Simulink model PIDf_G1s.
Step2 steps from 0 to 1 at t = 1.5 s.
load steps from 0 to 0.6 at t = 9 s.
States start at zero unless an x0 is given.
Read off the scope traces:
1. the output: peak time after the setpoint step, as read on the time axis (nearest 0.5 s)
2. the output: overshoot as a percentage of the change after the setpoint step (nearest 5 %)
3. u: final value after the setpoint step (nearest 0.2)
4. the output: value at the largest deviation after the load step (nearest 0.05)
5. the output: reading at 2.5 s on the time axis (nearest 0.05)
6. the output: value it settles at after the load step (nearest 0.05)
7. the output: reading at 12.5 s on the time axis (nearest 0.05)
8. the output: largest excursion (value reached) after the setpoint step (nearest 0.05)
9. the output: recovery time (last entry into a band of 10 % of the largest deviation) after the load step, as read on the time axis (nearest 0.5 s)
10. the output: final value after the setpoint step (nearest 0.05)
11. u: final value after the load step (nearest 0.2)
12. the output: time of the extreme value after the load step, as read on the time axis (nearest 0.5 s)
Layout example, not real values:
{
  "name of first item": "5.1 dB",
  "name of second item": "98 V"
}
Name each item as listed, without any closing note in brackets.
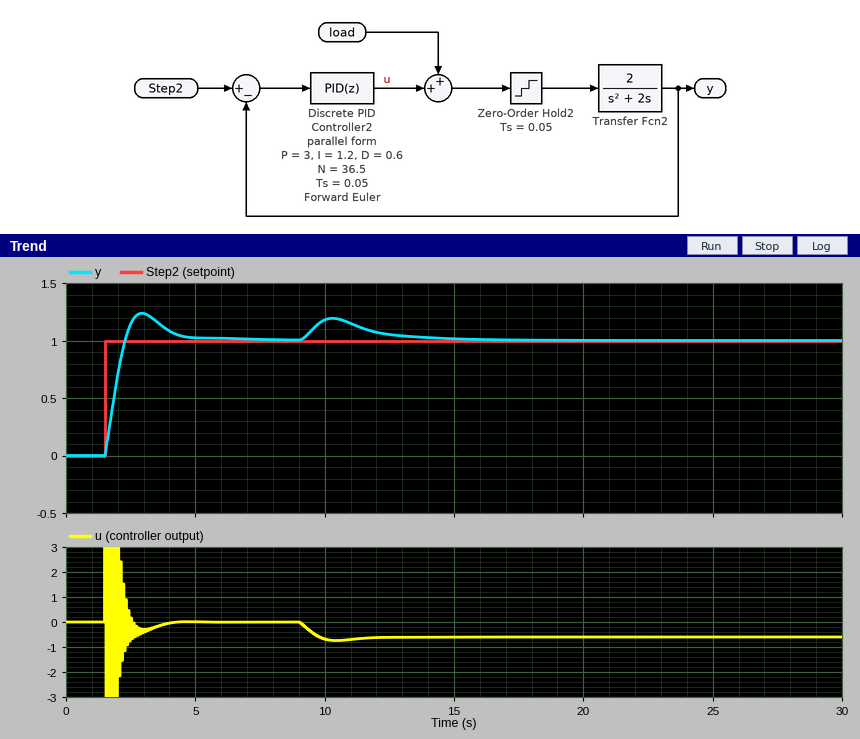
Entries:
{
  "the output: peak time after the setpoint step, as read on the time axis": "3.0 s",
  "the output: overshoot as a percentage of the change after the setpoint step": "25 %",
  "u: final value after the setpoint step": "0.0",
  "the output: value at the largest deviation after the load step": "1.20",
  "the output: reading at 2.5 s on the time axis": "1.15",
  "the output: value it settles at after the load step": "1.00",
  "the output: reading at 12.5 s on the time axis": "1.05",
  "the output: largest excursion (value reached) after the setpoint step": "1.25",
  "the output: recovery time (last entry into a band of 10 % of the largest deviation) after the load step, as read on the time axis": "14.5 s",
  "the output: final value after the setpoint step": "1.00",
  "u: final value after the load step": "-0.6",
  "the output: time of the extreme value after the load step, as read on the time axis": "10.5 s"
}
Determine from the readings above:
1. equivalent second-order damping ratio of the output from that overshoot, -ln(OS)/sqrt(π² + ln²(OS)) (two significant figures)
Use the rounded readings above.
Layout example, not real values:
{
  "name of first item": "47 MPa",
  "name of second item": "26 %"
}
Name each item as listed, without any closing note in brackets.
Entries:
{
  "equivalent second-order damping ratio of the output from that overshoot, -ln(OS)/sqrt(π² + ln²(OS))": "0.40"
}
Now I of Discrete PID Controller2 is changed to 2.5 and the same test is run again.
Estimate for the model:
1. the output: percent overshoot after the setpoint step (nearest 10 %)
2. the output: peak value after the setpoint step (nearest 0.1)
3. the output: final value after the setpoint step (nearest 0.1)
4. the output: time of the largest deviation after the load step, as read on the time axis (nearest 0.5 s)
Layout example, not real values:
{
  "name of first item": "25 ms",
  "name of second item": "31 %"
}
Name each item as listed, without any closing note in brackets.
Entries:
{
  "the output: percent overshoot after the setpoint step": "40 %",
  "the output: peak value after the setpoint step": "1.4",
  "the output: final value after the setpoint step": "1.0",
  "the output: time of the largest deviation after the load step, as read on the time axis": "10.0 s"
}
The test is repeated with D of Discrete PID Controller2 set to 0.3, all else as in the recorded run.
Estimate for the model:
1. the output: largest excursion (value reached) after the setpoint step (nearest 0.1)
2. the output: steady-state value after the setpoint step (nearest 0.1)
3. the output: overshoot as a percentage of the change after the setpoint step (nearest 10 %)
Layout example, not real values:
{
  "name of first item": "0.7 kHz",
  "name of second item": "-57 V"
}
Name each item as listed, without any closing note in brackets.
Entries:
{
  "the output: largest excursion (value reached) after the setpoint step": "1.3",
  "the output: steady-state value after the setpoint step": "1.0",
  "the output: overshoot as a percentage of the change after the setpoint step": "30 %"
}
